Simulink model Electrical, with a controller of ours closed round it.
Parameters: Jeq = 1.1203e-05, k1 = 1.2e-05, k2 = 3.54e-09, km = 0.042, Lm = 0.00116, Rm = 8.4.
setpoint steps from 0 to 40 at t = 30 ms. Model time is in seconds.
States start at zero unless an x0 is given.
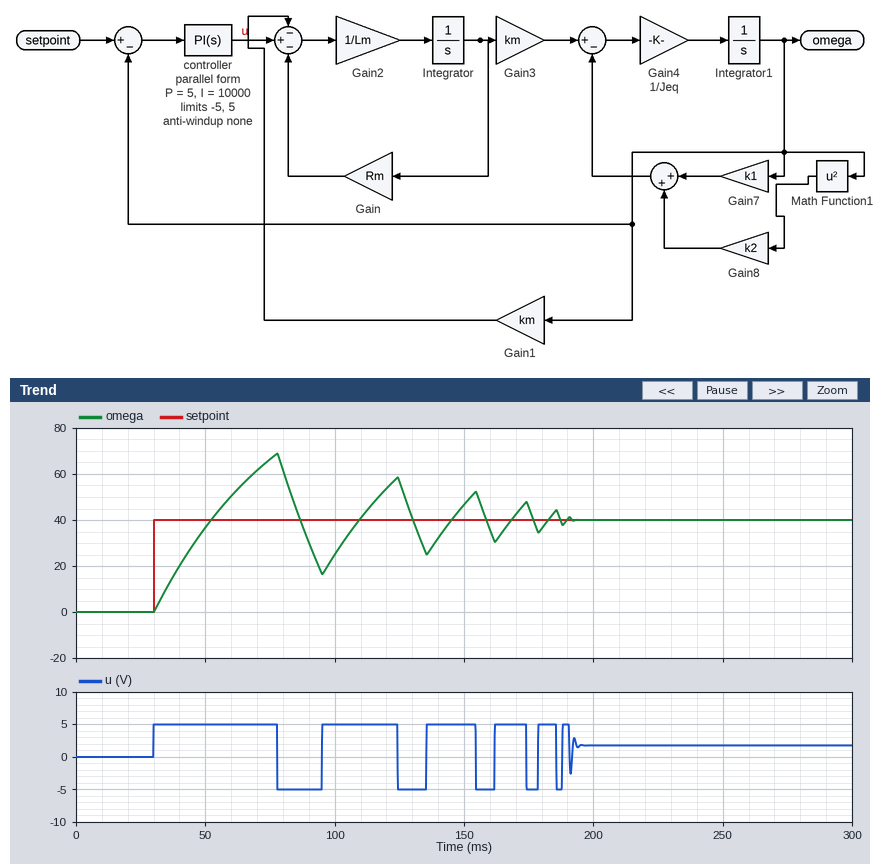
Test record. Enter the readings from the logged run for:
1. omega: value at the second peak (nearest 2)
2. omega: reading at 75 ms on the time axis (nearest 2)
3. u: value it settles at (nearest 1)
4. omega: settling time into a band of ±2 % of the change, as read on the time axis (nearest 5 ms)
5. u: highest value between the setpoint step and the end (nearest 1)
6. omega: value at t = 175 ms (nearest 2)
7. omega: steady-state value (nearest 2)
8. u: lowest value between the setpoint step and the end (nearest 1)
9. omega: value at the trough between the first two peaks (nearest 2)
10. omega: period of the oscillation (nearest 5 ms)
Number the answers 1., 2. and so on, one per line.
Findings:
1. 58
2. 66
3. 2
4. 190 ms
5. 5
6. 46
7. 40
8. -5
9. 16
10. 45 ms
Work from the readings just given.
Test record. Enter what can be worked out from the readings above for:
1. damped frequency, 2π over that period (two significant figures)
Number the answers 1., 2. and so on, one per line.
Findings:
1. 0.14 rad/ms
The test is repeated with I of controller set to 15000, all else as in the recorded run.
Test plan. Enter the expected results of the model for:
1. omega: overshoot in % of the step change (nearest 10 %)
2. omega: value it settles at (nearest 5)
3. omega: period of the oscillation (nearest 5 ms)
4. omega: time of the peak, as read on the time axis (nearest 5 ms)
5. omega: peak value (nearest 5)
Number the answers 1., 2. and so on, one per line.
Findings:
1. 70 %
2. 40
3. 50 ms
4. 80 ms
5. 70
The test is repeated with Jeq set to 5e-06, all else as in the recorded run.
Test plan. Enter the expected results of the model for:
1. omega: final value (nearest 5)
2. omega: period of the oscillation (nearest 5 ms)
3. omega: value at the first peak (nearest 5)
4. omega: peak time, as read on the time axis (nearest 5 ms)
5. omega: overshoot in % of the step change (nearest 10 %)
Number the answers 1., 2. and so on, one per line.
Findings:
1. 40
2. 20 ms
3. 70
4. 50 ms
5. 70 %
